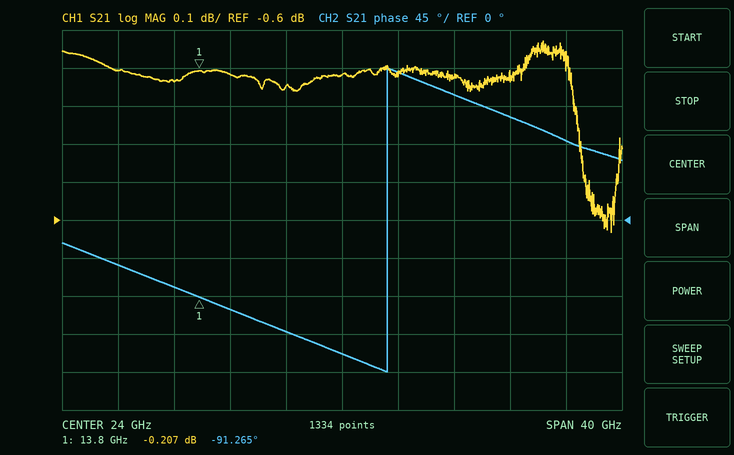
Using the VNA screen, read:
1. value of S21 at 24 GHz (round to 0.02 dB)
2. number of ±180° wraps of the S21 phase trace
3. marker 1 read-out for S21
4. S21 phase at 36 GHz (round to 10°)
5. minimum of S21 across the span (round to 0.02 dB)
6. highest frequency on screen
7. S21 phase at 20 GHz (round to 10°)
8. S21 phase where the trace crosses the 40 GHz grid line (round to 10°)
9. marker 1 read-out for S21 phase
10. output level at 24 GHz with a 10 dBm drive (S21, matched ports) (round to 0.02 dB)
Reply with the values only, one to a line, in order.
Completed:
-0.22 dB
1
-0.207 dB
120°
-0.64 dB
44 GHz
-130°
90°
-91.265°
9.78 dBm
